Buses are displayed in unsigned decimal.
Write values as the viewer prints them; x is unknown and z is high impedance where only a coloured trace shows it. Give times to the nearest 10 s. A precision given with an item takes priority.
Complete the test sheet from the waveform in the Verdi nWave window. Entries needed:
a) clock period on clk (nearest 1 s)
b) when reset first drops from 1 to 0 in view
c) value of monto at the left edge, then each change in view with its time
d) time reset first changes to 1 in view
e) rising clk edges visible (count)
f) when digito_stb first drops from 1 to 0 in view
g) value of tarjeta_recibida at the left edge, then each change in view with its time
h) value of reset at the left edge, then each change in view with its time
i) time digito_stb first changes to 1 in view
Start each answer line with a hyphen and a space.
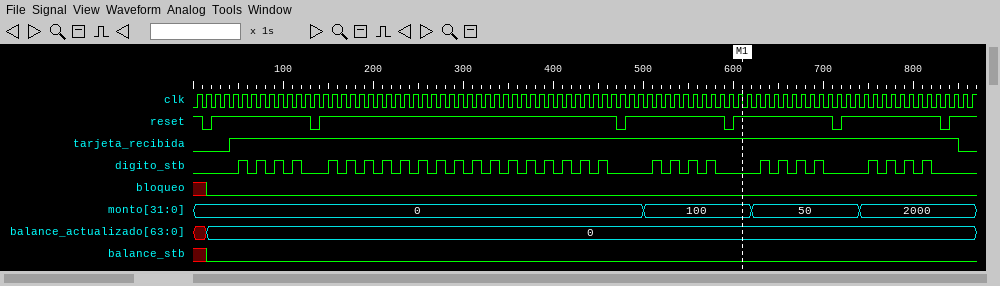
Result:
- 10 s
- 10 s
- 0, 100 at 500 s, 50 at 620 s, 2000 at 740 s
- 20 s
- 87
- 60 s
- 0, 1 at 40 s, 0 at 850 s
- 1, 0 at 10 s, 1 at 20 s, 0 at 130 s, 1 at 140 s, 0 at 470 s, 1 at 480 s, 0 at 590 s, 1 at 600 s, 0 at 710 s, 1 at 720 s, 0 at 830 s, 1 at 840 s
- 50 s
